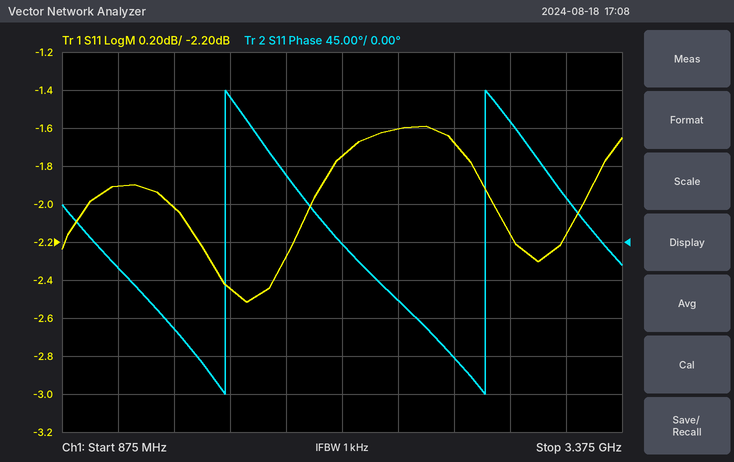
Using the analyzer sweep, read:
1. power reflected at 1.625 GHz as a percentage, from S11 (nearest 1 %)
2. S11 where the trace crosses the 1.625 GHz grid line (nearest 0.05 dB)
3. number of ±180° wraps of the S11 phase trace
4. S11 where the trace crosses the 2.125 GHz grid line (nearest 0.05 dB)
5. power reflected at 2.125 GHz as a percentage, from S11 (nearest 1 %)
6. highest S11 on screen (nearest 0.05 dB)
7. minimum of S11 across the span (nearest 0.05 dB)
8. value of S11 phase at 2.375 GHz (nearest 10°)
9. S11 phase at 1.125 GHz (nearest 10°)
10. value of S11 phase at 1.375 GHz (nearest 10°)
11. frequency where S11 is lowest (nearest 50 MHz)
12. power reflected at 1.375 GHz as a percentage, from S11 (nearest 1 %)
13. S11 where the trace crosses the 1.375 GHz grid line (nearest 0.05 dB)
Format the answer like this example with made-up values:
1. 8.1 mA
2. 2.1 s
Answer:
1. 57 %
2. -2.45 dB
3. 2
4. -1.75 dB
5. 67 %
6. -1.60 dB
7. -2.50 dB
8. -70°
9. -30°
10. -100°
11. 1.70 GHz
12. 63 %
13. -2.00 dB
